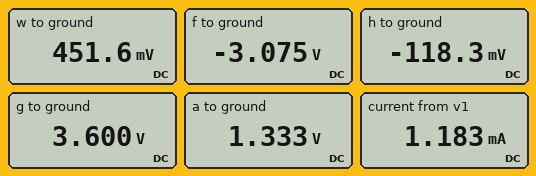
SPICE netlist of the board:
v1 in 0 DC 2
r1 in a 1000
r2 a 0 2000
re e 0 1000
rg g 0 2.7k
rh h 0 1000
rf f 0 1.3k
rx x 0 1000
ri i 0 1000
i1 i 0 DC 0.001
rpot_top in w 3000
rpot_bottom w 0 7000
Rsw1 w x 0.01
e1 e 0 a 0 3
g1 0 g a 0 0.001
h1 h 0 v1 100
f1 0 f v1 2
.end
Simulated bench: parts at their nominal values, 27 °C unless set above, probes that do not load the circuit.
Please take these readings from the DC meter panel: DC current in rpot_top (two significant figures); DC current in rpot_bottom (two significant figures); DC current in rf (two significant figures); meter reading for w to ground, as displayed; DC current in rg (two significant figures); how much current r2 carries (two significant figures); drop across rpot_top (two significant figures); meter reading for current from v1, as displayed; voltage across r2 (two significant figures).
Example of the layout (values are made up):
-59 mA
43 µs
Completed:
520 µA
65 µA
2.4 mA
451.6 mV
1.3 mA
670 µA
1.5 V
1.183 mA
1.3 V
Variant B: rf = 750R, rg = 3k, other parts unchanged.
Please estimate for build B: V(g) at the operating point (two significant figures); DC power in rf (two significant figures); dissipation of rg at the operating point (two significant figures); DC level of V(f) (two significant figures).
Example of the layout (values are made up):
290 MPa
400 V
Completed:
4.0 V
4.2 mW
5.3 mW
-1.8 V
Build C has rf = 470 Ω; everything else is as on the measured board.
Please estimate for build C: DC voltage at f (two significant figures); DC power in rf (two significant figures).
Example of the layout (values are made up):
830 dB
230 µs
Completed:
-1.1 V
2.6 mW
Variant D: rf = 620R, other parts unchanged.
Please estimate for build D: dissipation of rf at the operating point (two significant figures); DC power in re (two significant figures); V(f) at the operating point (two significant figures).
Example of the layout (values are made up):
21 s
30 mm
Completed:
3.5 mW
16 mW
-1.5 V
